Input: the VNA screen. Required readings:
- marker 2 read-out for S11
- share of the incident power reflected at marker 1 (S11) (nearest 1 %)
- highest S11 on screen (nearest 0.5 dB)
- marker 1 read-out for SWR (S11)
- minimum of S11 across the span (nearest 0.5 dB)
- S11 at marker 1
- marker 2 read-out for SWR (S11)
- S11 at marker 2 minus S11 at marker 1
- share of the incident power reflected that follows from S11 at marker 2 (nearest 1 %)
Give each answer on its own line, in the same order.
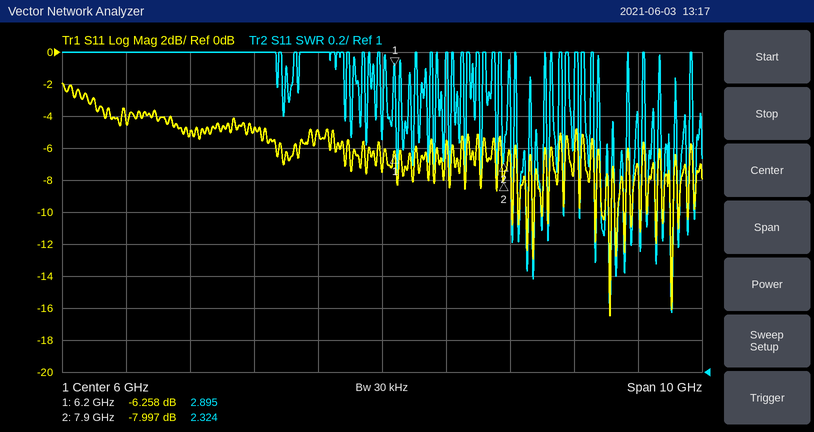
-7.997 dB
24 %
-2.0 dB
2.895
-16.5 dB
-6.258 dB
2.324
-1.739 dB
16 %
